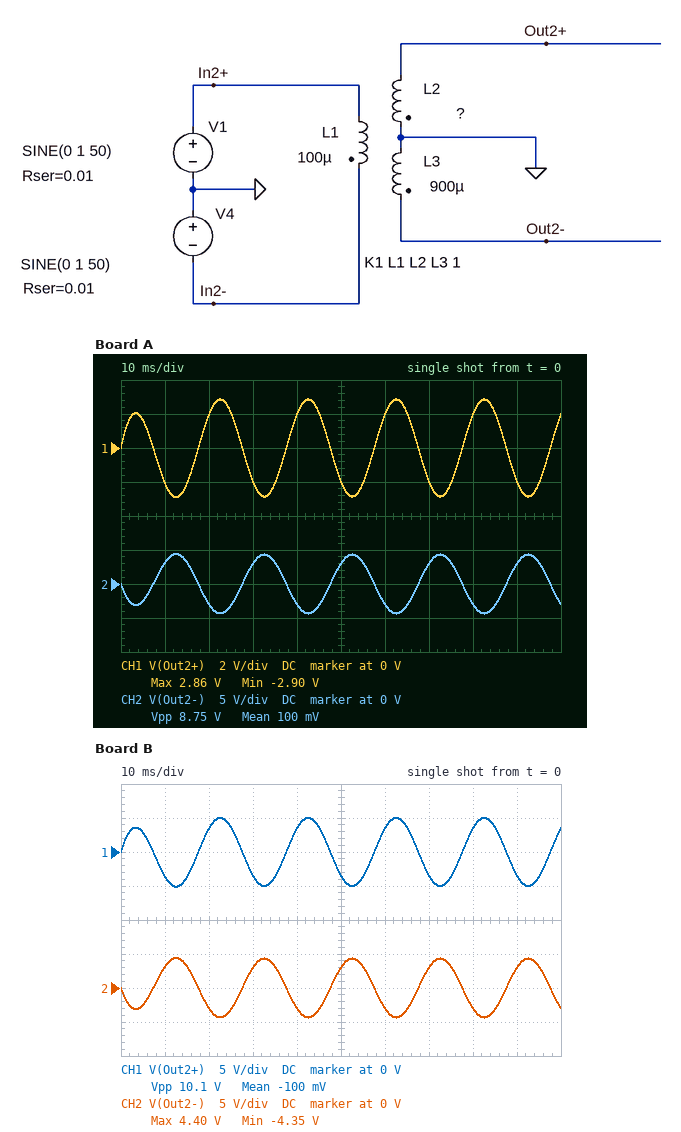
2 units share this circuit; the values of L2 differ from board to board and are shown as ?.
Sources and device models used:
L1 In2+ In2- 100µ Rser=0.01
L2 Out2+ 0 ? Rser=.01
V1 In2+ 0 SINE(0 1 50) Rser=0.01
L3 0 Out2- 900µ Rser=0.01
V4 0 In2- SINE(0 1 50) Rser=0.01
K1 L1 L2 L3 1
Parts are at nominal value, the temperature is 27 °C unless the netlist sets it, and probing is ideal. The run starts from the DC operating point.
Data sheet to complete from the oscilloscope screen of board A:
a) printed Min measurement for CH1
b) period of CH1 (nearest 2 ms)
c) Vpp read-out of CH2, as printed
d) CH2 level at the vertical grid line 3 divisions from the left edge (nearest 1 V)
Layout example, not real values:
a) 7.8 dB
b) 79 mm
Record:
a) -2.90 V
b) 20 ms
c) 8.75 V
d) 3 V
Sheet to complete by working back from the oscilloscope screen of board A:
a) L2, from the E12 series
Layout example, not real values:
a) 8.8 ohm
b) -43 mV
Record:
a) 390 µH
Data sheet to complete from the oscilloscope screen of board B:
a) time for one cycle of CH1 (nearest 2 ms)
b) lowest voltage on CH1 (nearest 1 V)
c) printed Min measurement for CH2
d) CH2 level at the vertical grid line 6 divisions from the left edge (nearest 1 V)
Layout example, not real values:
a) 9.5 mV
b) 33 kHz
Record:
a) 20 ms
b) -5 V
c) -4.35 V
d) -3 V
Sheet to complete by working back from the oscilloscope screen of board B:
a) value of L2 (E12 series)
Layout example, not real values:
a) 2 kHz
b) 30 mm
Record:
a) 1.2 mH
